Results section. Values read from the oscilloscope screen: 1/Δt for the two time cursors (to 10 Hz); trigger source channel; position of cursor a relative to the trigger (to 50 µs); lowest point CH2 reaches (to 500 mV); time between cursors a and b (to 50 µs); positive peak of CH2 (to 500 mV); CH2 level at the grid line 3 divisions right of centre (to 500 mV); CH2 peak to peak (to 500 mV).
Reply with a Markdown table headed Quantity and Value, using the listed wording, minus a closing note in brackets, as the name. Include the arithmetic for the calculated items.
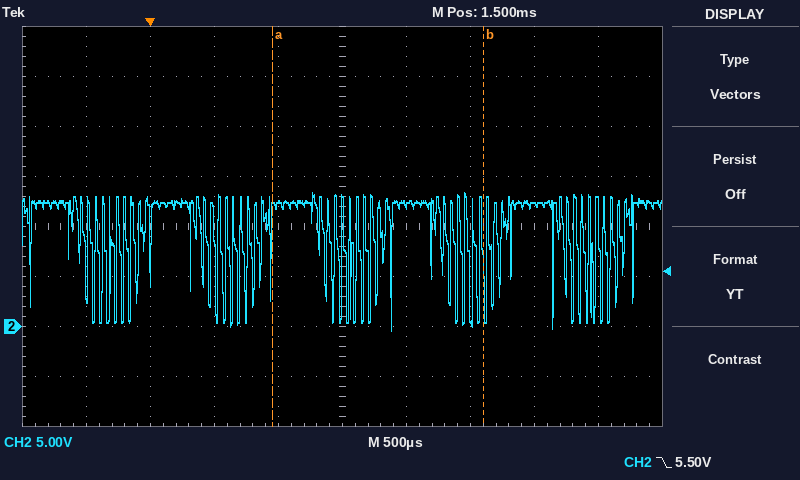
| Quantity | Value |
|---|---|
| 1/Δt for the two time cursors | 1 / 1.65 ms ≈ 610 Hz |
| trigger source channel | CH2 |
| position of cursor a relative to the trigger | +950 µs |
| lowest point CH2 reaches | -500 mV |
| time between cursors a and b | 1.65 ms |
| positive peak of CH2 | 13.5 V |
| CH2 level at the grid line 3 divisions right of centre | 12.0 V |
| CH2 peak to peak | 13.5 V − (-500 mV) = 14.0 V |
